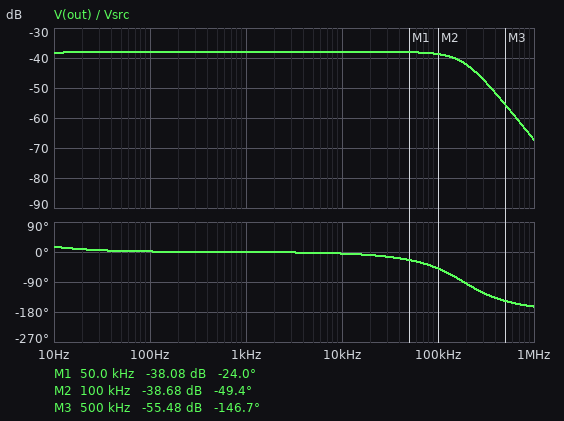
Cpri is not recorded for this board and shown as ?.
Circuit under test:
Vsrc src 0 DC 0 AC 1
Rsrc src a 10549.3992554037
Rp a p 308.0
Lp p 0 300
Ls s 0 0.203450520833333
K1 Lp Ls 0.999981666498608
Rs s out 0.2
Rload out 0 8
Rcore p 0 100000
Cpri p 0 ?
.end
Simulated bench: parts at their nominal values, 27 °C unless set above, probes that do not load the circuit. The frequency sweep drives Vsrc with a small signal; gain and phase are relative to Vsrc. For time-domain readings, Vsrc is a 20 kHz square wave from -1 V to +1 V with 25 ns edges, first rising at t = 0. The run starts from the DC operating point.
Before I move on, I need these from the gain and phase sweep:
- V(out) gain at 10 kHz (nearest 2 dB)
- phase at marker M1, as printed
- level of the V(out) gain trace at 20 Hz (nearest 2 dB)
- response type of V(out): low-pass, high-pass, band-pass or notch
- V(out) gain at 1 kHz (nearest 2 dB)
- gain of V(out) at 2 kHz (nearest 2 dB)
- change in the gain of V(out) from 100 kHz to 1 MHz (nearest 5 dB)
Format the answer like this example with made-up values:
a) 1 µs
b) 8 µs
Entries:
a) -38 dB
b) -24.0 deg
c) -38 dB
d) low-pass
e) -38 dB
f) -38 dB
g) -30 dB
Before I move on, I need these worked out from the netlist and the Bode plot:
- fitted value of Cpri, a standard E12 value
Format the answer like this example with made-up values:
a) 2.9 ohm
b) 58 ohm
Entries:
a) 150 pF
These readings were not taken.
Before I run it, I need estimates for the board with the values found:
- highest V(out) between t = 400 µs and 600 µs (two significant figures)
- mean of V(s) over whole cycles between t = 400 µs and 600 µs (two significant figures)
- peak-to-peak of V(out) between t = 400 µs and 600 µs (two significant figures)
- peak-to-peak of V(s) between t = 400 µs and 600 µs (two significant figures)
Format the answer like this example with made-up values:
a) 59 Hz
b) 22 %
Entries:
a) 26 mV
b) 13 mV
c) 27 mV
d) 27 mV
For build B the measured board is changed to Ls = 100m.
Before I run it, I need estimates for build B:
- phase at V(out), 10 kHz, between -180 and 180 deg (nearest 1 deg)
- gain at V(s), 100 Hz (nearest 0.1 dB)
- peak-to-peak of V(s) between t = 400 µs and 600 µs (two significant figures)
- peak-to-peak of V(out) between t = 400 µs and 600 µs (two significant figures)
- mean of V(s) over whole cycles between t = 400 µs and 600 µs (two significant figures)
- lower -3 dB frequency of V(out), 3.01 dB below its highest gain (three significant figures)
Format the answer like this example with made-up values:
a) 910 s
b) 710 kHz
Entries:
a) -5 deg
b) -38.6 dB
c) 24 mV
d) 23 mV
e) 12 mV
f) 3.72 Hz
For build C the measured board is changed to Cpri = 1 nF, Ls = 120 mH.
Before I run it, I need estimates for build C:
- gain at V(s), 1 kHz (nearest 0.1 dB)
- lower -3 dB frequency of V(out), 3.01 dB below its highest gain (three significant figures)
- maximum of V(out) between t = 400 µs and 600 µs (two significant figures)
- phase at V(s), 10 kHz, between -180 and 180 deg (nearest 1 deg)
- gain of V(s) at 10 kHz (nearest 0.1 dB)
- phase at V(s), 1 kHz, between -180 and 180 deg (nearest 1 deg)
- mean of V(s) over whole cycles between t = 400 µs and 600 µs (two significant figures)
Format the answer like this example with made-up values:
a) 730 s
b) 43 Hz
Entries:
a) -38.3 dB
b) 3.52 Hz
c) 23 mV
d) -24 deg
e) -38.9 dB
f) -2 deg
g) 12 mV
